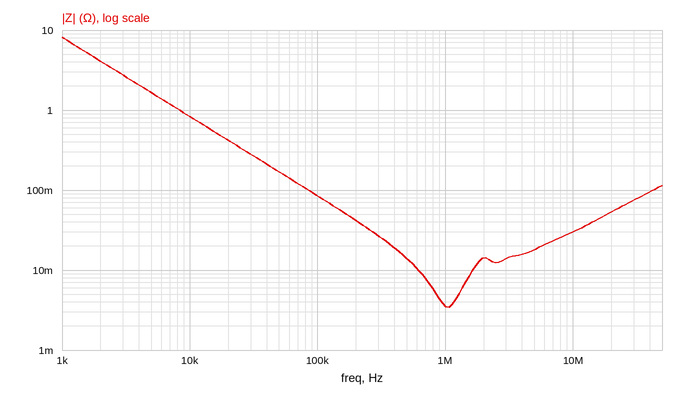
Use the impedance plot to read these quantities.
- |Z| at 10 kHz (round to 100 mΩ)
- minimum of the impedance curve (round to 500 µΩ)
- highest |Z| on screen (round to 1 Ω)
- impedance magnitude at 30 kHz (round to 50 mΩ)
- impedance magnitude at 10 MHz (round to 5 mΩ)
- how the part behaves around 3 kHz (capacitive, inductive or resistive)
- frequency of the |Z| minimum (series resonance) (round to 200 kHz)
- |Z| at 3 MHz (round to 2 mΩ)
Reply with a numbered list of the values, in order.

1. 800 mΩ
2. 3.5 mΩ
3. 8 Ω
4. 300 mΩ
5. 30 mΩ
6. capacitive
7. 1.0 MHz
8. 14 mΩ
